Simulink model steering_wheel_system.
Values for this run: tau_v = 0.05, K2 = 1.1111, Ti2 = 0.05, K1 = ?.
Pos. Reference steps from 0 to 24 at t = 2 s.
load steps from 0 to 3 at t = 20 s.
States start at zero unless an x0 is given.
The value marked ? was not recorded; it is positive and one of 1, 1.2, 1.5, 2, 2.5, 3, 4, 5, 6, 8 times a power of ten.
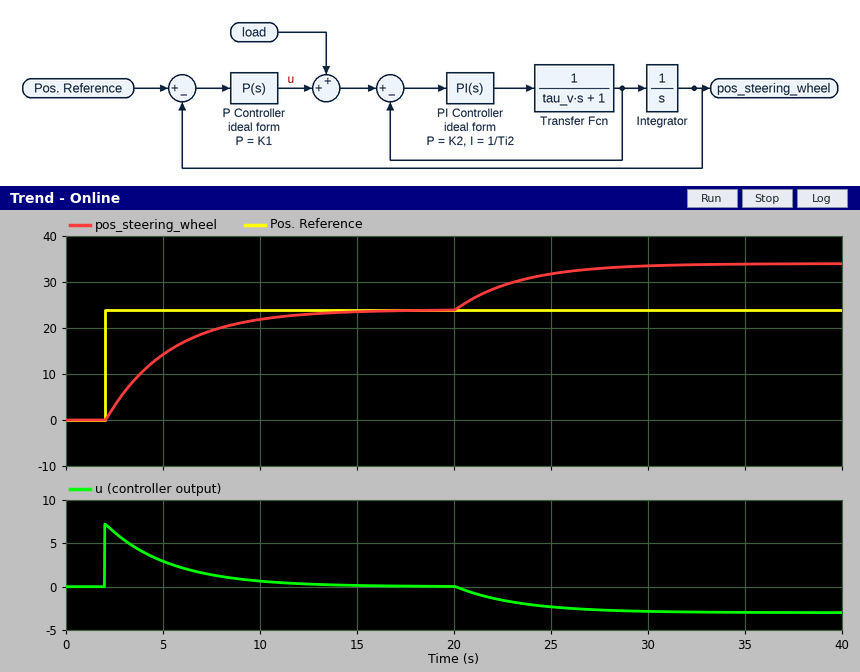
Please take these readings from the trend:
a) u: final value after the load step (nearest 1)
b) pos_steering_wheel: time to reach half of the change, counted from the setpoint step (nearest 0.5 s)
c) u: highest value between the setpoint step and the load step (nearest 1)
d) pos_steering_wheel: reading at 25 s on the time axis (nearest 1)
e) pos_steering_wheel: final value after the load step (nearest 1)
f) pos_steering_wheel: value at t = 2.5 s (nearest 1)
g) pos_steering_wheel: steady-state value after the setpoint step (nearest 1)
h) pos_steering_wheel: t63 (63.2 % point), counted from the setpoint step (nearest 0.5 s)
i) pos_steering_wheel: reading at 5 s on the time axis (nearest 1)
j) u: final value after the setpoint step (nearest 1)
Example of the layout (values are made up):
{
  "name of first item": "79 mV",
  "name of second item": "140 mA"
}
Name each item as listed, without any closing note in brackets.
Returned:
{
  "u: final value after the load step": "-3",
  "pos_steering_wheel: time to reach half of the change, counted from the setpoint step": "2.5 s",
  "u: highest value between the setpoint step and the load step": "7",
  "pos_steering_wheel: reading at 25 s on the time axis": "32",
  "pos_steering_wheel: final value after the load step": "34",
  "pos_steering_wheel: value at t = 2.5 s": "3",
  "pos_steering_wheel: steady-state value after the setpoint step": "24",
  "pos_steering_wheel: t63 (63.2 % point), counted from the setpoint step": "3.5 s",
  "pos_steering_wheel: reading at 5 s on the time axis": "14",
  "u: final value after the setpoint step": "0"
}
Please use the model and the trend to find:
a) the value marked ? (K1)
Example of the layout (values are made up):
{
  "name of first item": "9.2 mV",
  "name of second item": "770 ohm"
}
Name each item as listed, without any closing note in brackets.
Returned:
{
  "the value marked ?": "0.3"
}
